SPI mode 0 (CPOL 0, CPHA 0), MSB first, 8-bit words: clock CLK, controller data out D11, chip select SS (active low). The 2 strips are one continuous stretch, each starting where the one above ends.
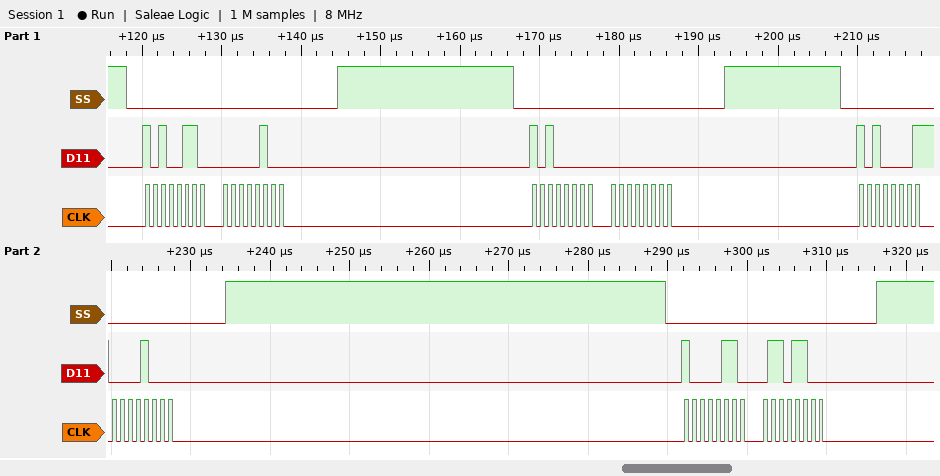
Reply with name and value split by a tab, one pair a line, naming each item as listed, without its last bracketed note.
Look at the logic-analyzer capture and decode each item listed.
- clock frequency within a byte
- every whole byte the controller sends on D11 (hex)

clock frequency within a byte	1 MHz
every whole byte the controller sends on D11	0xA6 0x04 0xA0 0x00 0xA1 0x08 0x86 0x6C
